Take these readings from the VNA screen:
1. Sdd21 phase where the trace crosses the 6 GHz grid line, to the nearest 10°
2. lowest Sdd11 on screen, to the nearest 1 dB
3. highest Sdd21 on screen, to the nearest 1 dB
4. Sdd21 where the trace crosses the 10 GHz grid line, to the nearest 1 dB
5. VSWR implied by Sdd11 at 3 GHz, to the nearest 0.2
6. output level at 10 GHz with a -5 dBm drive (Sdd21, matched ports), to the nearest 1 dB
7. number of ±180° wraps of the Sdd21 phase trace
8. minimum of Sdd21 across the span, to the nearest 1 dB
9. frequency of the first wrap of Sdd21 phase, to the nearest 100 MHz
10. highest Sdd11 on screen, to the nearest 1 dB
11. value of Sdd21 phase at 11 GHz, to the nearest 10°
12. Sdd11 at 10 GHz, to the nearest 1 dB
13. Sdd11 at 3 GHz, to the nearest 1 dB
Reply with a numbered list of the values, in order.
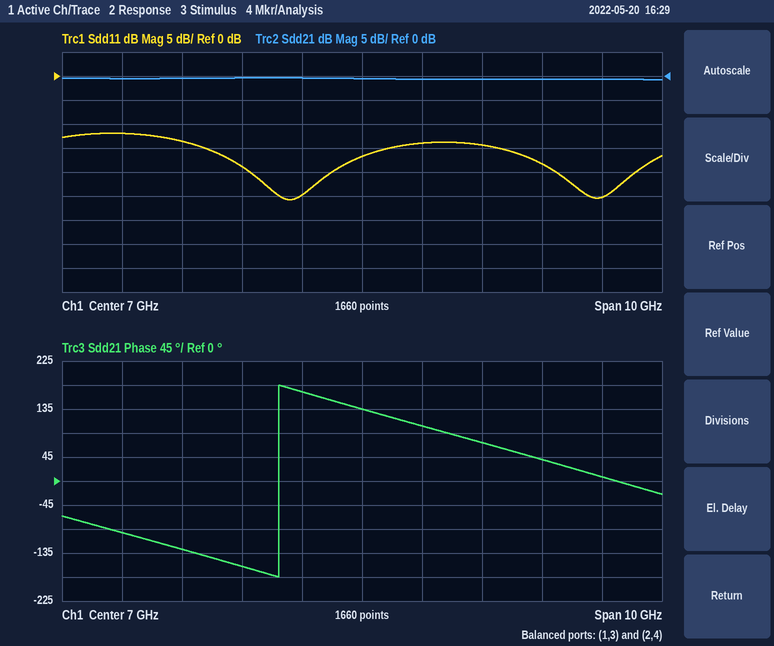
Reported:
1. 170°
2. -26 dB
3. 0 dB
4. -1 dB
5. 1.6
6. -6 dBm
7. 1
8. -1 dB
9. 5.6 GHz
10. -12 dB
11. 10°
12. -18 dB
13. -12 dB
